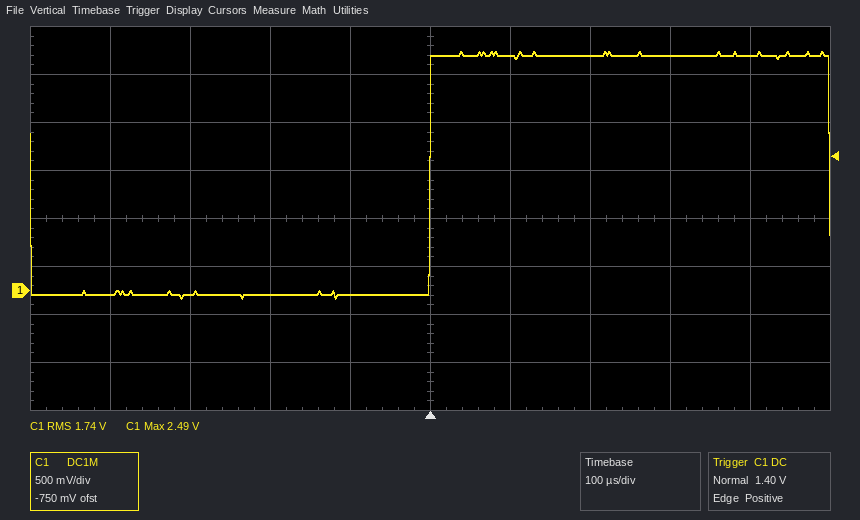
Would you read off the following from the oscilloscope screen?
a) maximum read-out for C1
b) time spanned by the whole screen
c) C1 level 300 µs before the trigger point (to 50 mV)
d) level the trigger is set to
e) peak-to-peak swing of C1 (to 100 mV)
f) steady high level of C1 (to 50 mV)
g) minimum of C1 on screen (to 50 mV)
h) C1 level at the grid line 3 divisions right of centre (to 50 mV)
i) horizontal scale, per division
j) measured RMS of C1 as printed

2.49 V
1 ms
-50 mV
1.40 V
2.60 V
2.45 V
-100 mV
2.45 V
100 µs
1.74 V
